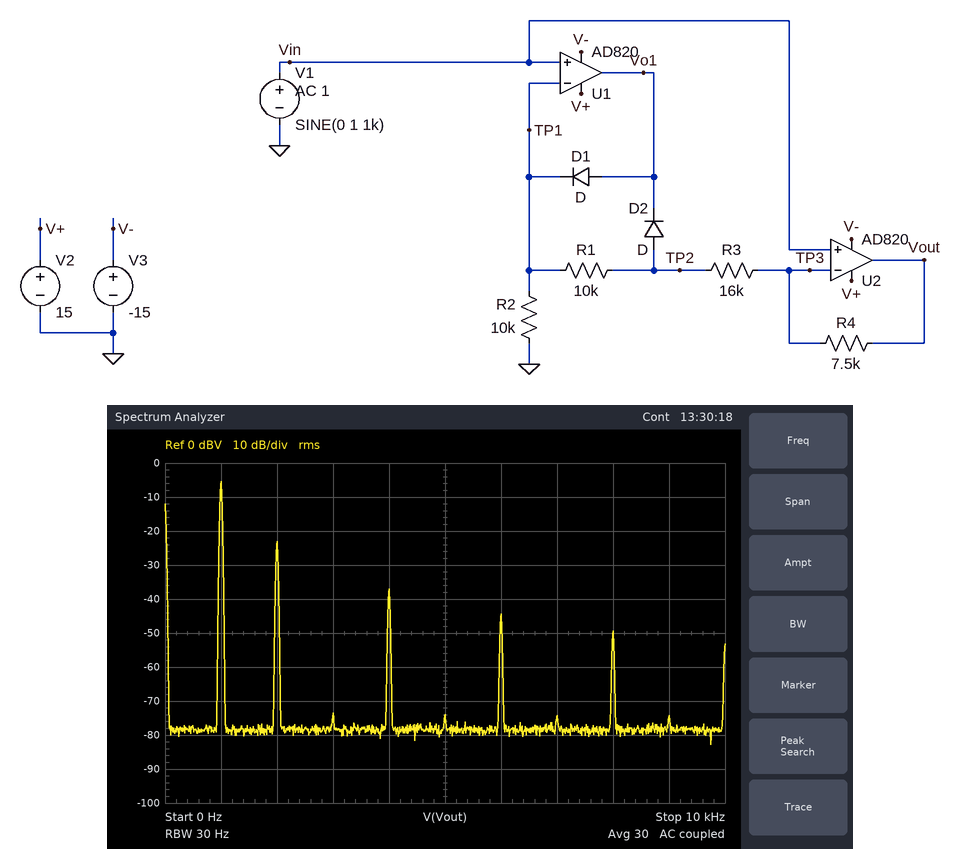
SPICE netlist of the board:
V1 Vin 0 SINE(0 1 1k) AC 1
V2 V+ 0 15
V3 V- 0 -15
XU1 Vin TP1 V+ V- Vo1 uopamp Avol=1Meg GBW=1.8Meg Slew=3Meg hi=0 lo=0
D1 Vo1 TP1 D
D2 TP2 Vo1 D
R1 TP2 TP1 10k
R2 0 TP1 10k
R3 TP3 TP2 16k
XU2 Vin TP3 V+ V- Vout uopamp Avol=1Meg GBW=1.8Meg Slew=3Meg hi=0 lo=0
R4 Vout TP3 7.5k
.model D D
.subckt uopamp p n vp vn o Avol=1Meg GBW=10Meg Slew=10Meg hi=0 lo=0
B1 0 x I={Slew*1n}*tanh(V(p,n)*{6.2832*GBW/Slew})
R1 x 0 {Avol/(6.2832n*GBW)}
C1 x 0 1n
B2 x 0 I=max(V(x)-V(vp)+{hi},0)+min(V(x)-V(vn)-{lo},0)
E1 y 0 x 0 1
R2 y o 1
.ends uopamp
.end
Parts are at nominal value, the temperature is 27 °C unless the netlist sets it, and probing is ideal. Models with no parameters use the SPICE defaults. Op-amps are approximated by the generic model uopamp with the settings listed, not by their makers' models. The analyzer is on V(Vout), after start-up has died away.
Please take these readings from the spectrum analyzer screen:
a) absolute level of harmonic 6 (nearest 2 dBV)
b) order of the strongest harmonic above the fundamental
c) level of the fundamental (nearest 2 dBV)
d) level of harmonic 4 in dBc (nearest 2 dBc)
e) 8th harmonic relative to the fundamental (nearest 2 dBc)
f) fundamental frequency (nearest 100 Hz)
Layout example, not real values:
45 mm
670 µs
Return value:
-44 dBV
2
-6 dBV
-32 dBc
-44 dBc
1.0 kHz
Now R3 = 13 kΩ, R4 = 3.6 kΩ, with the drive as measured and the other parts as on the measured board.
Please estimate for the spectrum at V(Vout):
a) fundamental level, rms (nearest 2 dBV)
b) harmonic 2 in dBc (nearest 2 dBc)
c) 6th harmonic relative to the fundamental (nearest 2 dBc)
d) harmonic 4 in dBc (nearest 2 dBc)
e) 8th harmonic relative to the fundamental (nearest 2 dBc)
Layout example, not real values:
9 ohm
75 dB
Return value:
-4 dBV
-24 dBc
-44 dBc
-38 dBc
-50 dBc
